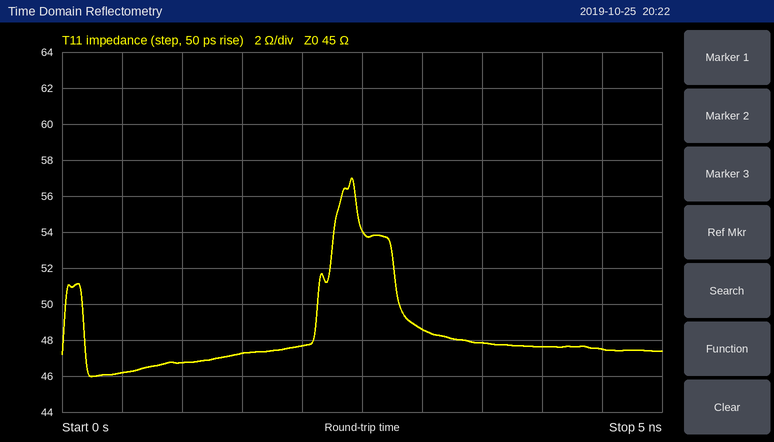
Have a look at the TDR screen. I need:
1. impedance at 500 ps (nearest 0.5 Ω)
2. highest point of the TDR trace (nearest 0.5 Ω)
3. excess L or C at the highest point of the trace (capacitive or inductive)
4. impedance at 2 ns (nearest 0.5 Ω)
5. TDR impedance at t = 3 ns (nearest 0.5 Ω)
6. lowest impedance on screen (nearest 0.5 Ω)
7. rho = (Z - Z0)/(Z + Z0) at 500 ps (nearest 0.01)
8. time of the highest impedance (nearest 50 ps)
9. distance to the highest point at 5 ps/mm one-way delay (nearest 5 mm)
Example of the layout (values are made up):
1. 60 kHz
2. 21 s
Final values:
1. 46.0 Ω
2. 57.0 Ω
3. inductive
4. 47.5 Ω
5. 48.5 Ω
6. 46.0 Ω
7. +0.01
8. 2.40 ns
9. 240 mm
